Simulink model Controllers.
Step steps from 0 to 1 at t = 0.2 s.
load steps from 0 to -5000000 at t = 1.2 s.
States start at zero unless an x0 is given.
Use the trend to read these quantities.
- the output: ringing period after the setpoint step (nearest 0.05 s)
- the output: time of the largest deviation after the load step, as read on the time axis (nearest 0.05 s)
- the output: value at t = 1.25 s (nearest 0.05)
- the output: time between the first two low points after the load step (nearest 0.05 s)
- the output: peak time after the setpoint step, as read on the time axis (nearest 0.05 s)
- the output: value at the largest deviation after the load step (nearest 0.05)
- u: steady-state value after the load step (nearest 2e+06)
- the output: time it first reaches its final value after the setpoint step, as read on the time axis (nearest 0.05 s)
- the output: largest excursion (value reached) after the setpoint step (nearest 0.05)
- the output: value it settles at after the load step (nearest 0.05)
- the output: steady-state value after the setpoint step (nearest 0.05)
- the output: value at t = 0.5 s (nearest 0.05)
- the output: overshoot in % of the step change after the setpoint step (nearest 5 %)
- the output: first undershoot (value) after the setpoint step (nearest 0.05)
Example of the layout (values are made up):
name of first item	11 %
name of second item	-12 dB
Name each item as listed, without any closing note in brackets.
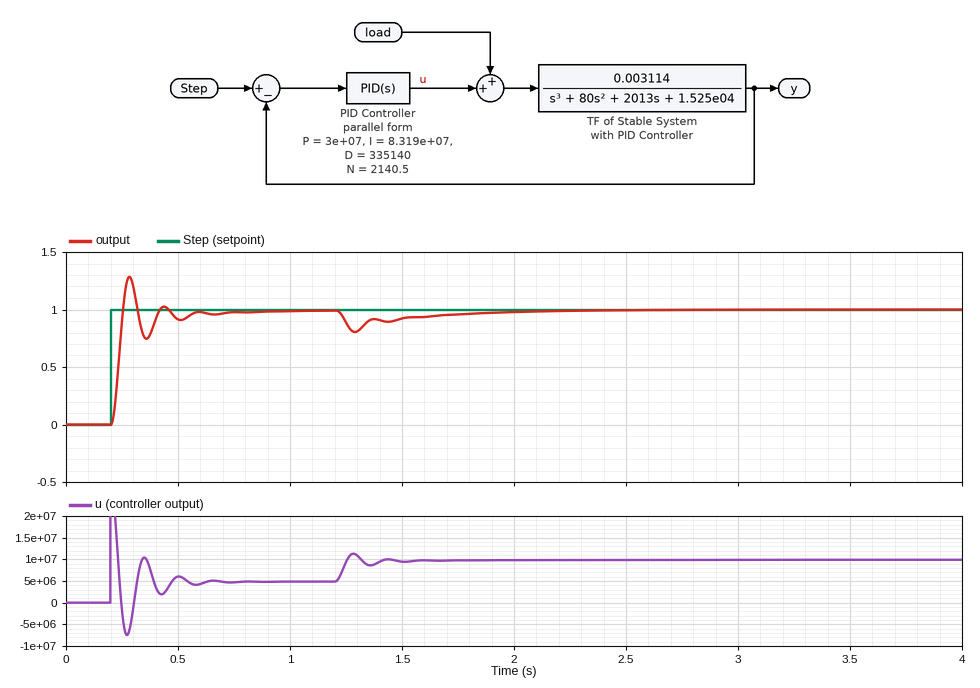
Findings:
the output: ringing period after the setpoint step	0.15 s
the output: time of the largest deviation after the load step, as read on the time axis	1.30 s
the output: value at t = 1.25 s	0.90
the output: time between the first two low points after the load step	0.15 s
the output: peak time after the setpoint step, as read on the time axis	0.30 s
the output: value at the largest deviation after the load step	0.80
u: steady-state value after the load step	10000000
the output: time it first reaches its final value after the setpoint step, as read on the time axis	0.25 s
the output: largest excursion (value reached) after the setpoint step	1.30
the output: value it settles at after the load step	1.00
the output: steady-state value after the setpoint step	1.00
the output: value at t = 0.5 s	0.90
the output: overshoot in % of the step change after the setpoint step	30 %
the output: first undershoot (value) after the setpoint step	0.75
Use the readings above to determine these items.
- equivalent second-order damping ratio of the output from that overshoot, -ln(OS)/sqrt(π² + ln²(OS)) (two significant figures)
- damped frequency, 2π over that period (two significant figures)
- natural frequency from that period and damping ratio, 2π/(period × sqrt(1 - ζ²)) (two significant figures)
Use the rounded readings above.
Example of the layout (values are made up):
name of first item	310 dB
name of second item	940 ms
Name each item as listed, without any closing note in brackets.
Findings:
equivalent second-order damping ratio of the output from that overshoot, -ln(OS)/sqrt(π² + ln²(OS))	0.36
damped frequency, 2π over that period	42 rad/s
natural frequency from that period and damping ratio, 2π/(period × sqrt(1 - ζ²))	45 rad/s
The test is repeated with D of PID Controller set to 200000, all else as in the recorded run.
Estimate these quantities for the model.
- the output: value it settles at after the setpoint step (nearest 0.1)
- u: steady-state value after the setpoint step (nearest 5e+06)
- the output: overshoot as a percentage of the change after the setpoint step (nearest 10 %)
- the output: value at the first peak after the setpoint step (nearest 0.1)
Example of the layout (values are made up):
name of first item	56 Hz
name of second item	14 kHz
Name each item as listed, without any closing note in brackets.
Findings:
the output: value it settles at after the setpoint step	1.0
u: steady-state value after the setpoint step	5000000
the output: overshoot as a percentage of the change after the setpoint step	40 %
the output: value at the first peak after the setpoint step	1.4
